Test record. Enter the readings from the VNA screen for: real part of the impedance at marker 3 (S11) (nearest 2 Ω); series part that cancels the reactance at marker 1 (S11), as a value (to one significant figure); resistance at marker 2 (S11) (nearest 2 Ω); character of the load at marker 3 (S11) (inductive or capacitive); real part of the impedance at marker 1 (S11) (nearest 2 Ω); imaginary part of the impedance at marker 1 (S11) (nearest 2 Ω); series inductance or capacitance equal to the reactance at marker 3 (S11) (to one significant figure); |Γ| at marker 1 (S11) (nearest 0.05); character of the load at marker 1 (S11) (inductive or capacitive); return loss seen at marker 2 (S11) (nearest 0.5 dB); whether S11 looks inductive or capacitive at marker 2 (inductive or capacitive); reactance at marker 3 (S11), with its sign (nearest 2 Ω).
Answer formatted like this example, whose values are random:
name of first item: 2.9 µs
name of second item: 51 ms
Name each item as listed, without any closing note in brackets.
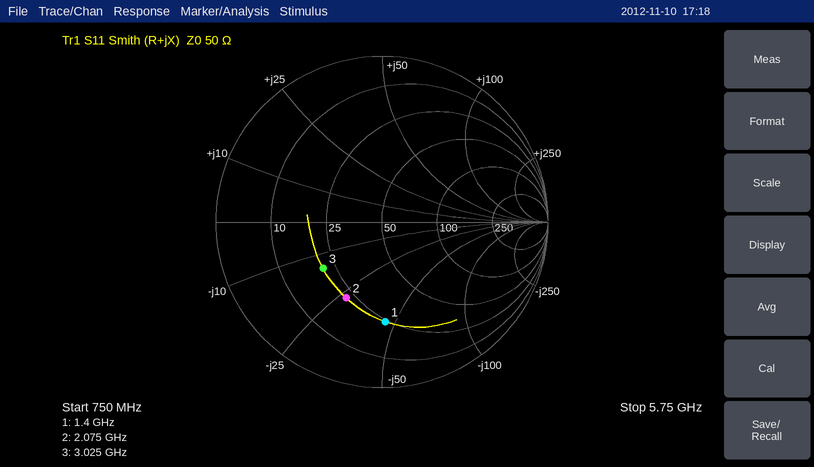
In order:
real part of the impedance at marker 3 (S11): 20 Ω
series part that cancels the reactance at marker 1 (S11), as a value: 5 nH
resistance at marker 2 (S11): 22 Ω
character of the load at marker 3 (S11): capacitive
real part of the impedance at marker 1 (S11): 24 Ω
imaginary part of the impedance at marker 1 (S11): -46 Ω
series inductance or capacitance equal to the reactance at marker 3 (S11): 4 pF
|Γ| at marker 1 (S11): 0.60
character of the load at marker 1 (S11): capacitive
return loss seen at marker 2 (S11): 6.0 dB
whether S11 looks inductive or capacitive at marker 2: capacitive
reactance at marker 3 (S11), with its sign: -14 Ω
